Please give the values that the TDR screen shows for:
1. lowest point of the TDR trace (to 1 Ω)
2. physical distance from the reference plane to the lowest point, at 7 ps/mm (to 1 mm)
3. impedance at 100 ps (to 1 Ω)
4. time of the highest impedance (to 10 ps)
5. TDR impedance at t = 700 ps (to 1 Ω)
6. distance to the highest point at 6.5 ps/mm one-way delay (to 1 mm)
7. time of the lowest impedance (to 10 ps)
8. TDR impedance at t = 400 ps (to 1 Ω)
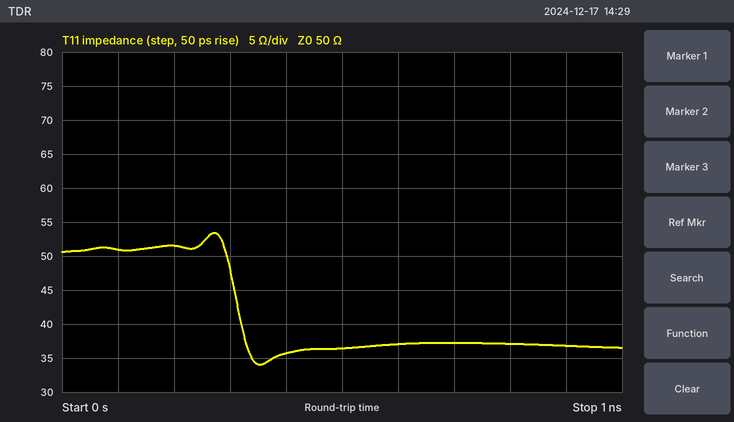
34 Ω
25 mm
51 Ω
270 ps
37 Ω
21 mm
350 ps
36 Ω
